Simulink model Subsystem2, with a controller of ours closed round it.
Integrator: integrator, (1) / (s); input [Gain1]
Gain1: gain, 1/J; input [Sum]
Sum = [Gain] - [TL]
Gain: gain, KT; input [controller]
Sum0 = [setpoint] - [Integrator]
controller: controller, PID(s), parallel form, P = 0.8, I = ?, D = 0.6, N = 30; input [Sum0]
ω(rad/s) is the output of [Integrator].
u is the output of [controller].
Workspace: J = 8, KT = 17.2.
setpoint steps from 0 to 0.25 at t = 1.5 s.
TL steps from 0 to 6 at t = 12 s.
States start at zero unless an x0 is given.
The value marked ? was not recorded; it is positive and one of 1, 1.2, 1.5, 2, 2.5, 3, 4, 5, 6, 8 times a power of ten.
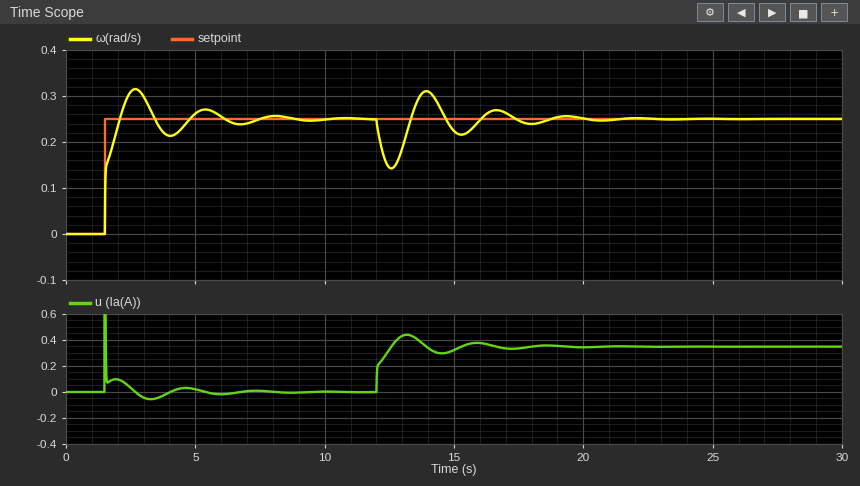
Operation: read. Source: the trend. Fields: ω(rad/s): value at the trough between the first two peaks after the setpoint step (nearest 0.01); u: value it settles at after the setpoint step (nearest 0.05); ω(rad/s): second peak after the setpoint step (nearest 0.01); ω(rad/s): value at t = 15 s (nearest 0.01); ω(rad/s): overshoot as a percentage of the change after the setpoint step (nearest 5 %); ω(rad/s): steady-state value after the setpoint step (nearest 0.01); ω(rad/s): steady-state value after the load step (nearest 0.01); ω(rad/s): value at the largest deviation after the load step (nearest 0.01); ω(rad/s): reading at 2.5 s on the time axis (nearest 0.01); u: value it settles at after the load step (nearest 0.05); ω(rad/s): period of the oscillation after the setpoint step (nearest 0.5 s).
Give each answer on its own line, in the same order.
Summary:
0.21
0.00
0.27
0.22
25 %
0.25
0.25
0.14
0.31
0.35
2.5 s
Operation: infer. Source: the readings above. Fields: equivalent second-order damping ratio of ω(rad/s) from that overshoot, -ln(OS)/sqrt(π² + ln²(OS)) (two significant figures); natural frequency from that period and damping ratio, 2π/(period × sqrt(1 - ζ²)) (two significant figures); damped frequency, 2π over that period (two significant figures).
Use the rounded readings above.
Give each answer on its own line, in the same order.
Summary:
0.40
2.7 rad/s
2.5 rad/s
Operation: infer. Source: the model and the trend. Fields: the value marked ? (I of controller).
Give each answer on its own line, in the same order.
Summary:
6
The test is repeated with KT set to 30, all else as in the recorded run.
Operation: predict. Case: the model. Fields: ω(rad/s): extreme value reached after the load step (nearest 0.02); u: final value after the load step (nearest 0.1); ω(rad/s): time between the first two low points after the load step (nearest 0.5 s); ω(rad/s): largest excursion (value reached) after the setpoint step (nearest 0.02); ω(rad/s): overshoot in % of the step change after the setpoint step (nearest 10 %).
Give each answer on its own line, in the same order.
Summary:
0.18
0.2
2.5 s
0.30
20 %
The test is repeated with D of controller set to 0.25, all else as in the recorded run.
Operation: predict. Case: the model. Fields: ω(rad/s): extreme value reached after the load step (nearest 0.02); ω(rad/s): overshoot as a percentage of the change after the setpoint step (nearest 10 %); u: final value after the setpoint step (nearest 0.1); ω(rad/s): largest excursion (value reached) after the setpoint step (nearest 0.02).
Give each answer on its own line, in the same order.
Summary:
0.12
40 %
0.0
0.34
